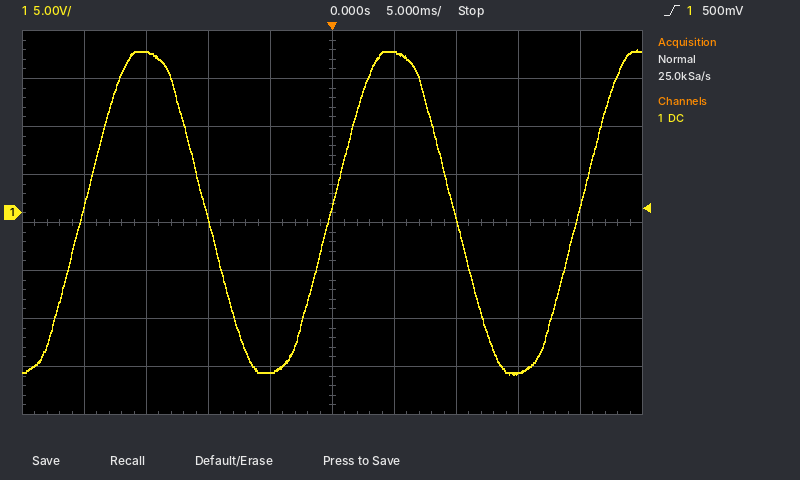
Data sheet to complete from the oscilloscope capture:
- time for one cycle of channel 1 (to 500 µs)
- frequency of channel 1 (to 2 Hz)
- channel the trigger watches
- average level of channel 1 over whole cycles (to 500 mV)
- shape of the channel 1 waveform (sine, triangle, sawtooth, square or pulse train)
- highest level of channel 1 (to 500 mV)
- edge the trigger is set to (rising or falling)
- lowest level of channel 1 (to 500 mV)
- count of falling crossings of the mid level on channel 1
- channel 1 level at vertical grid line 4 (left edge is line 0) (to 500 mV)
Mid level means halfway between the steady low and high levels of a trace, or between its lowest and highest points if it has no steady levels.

20.0 ms
50 Hz
channel 1
0.0 V
sine
17.0 V
rising
-17.0 V
2
-16.5 V
